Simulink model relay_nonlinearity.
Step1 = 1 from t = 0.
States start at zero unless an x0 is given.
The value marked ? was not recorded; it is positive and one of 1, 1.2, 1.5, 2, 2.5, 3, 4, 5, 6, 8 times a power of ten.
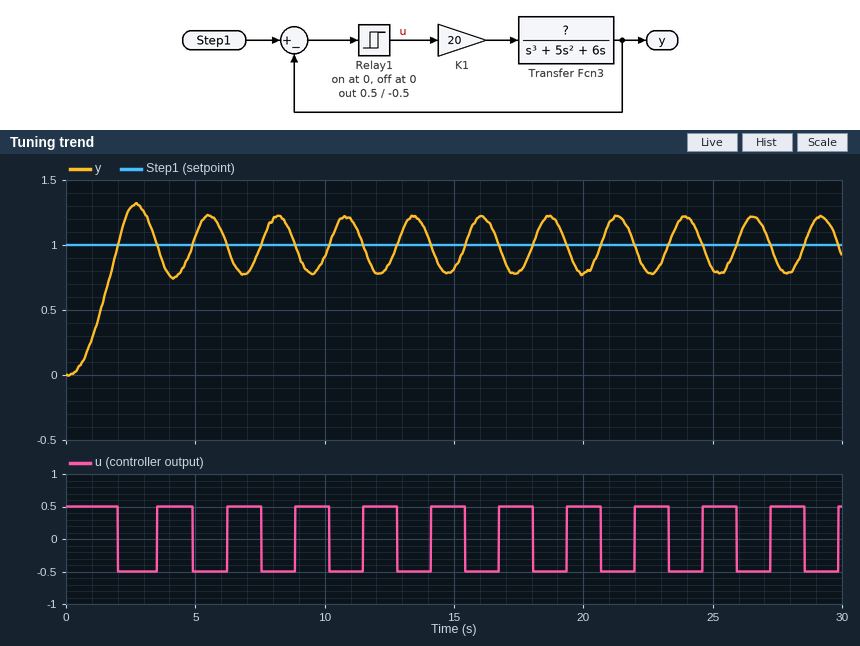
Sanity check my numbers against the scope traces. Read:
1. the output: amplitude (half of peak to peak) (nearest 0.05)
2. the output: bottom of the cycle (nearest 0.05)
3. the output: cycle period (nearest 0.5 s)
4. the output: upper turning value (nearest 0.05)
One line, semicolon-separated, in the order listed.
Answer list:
0.20; 0.80; 2.5 s; 1.20
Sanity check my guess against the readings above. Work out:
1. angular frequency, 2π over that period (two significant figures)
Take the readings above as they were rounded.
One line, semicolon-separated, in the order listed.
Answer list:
2.5 rad/s
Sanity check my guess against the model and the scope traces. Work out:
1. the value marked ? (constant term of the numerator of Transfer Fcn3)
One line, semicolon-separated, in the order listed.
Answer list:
0.5
